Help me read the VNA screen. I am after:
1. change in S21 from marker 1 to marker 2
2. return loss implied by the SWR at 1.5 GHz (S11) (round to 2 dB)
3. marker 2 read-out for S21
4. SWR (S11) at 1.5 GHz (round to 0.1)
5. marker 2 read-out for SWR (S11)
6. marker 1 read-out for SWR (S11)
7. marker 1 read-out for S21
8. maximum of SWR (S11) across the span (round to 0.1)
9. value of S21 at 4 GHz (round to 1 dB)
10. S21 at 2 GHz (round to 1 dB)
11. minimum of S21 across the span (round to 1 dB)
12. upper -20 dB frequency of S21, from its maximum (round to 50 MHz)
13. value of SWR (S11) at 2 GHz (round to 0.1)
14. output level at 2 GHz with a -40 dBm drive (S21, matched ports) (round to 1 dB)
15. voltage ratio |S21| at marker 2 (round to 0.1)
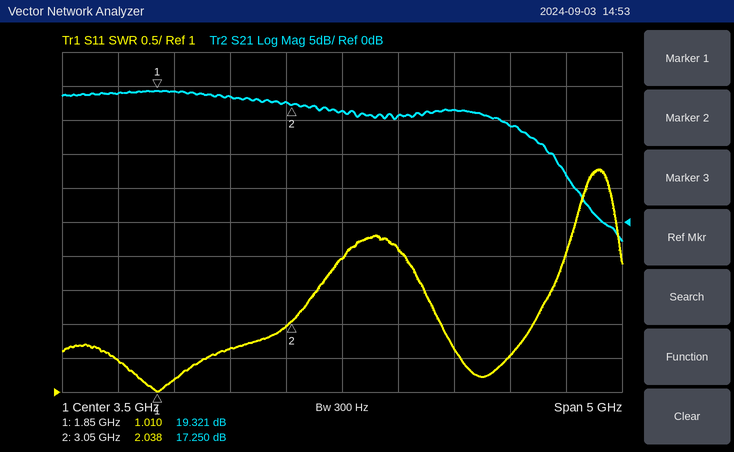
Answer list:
-2.071 dB
14 dB
17.250 dB
1.5
2.038
1.010
19.321 dB
4.3
16 dB
19 dB
-3 dB
5.90 GHz
1.2
-21 dBm
7.3
